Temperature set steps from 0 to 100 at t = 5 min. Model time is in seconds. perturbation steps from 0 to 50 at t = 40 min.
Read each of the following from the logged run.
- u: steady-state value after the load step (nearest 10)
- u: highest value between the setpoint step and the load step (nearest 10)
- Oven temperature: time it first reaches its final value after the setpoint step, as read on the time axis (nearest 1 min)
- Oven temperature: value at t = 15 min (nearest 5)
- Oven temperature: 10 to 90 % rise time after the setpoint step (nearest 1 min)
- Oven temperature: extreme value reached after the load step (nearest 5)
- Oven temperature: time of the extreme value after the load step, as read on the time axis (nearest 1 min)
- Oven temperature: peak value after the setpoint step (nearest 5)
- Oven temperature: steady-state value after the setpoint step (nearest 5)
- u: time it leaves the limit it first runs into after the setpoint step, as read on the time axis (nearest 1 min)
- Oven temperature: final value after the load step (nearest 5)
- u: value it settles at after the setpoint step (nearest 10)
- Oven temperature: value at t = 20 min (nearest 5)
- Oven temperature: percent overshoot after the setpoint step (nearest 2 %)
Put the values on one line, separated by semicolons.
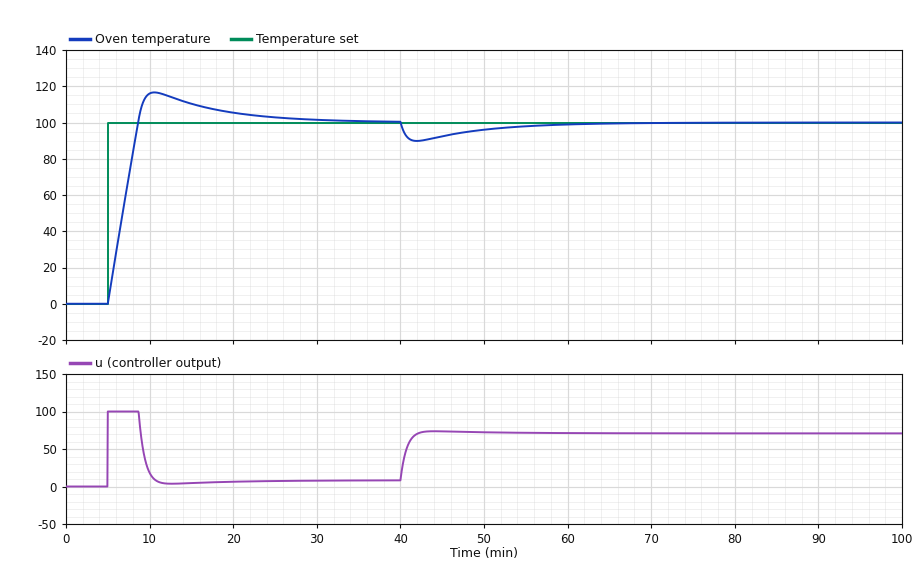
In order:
70; 100; 9 min; 110; 3 min; 90; 42 min; 115; 100; 9 min; 100; 10; 105; 16 %
